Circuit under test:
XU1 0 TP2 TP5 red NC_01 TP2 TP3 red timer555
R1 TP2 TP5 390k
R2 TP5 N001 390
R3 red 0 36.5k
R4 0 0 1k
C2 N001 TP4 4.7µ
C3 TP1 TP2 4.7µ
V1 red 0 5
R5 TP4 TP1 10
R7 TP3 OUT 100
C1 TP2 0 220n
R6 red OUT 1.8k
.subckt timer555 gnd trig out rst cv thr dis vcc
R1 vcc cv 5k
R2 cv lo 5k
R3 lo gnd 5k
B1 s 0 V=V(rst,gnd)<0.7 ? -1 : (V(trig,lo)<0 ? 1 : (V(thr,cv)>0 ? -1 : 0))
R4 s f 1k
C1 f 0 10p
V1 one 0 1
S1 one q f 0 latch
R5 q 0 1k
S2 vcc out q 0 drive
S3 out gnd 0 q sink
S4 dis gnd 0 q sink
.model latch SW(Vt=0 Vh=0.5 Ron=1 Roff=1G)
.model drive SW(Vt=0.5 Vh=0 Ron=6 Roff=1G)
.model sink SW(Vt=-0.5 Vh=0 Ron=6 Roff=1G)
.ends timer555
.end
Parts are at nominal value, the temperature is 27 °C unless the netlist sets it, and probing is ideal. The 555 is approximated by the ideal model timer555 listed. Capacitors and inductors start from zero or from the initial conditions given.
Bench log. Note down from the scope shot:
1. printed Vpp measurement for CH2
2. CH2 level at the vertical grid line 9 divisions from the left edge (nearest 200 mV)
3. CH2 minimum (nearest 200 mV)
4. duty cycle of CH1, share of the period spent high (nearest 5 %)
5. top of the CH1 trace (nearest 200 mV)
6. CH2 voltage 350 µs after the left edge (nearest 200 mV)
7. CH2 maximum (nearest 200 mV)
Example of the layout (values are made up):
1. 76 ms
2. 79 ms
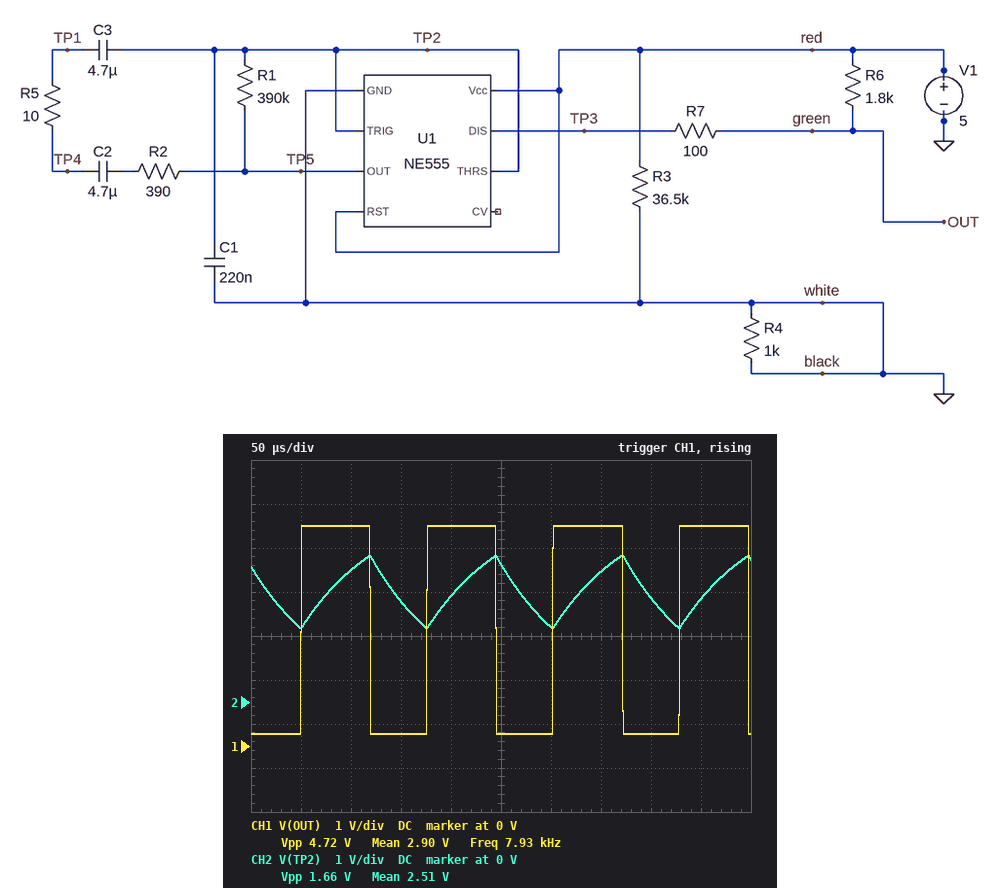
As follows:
1. 1.66 V
2. 2.4 V
3. 1.6 V
4. 55 %
5. 5.0 V
6. 3.0 V
7. 3.4 V
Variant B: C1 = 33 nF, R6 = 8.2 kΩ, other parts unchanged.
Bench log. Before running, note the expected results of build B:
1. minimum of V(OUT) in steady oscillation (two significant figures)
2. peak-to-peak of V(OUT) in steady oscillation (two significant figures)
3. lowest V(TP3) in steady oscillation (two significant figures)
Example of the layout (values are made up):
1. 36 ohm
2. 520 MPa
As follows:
1. 64 mV
2. 4.9 V
3. 3.6 mV
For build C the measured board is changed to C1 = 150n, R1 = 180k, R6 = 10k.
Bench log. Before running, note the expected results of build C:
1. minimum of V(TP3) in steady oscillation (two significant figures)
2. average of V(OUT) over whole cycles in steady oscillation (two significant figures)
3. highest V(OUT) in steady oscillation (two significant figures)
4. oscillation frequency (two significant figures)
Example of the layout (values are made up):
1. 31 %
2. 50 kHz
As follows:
1. 3.0 mV
2. 2.7 V
3. 5.0 V
4. 12 kHz
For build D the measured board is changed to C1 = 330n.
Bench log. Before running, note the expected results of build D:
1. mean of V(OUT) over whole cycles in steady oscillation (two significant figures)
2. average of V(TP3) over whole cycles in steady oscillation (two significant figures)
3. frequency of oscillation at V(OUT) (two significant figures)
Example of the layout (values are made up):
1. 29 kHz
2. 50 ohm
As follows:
1. 3.0 V
2. 2.9 V
3. 5.2 kHz
